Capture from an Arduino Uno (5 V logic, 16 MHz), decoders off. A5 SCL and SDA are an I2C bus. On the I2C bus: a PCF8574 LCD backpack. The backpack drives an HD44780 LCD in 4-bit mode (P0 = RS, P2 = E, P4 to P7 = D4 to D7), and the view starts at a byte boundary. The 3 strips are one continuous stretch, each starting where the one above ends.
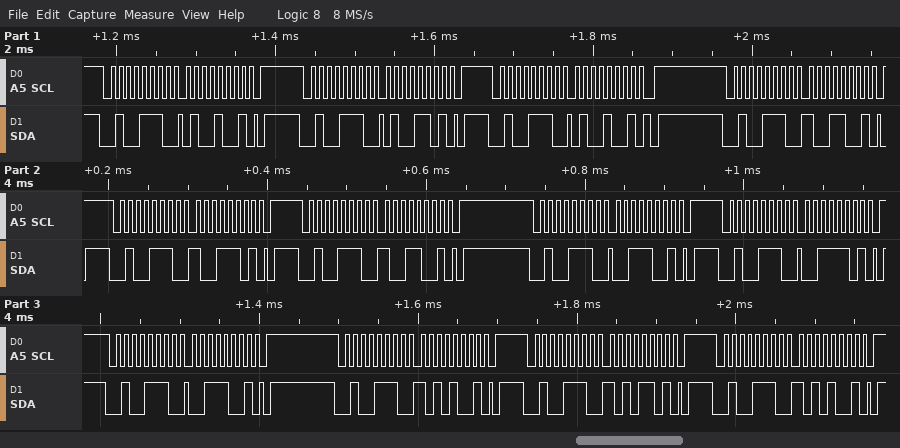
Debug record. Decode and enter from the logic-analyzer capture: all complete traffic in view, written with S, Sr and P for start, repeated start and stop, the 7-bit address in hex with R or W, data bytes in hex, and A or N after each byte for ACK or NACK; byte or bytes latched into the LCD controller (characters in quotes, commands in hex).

S 27W A 49 A P S 27W A 4D A P S 27W A 49 A P S 27W A 99 A P S 27W A 9D A P S 27W A 99 A P S 27W A 39 A P S 27W A 3D A P S 27W A 39 A P S 27W A A9 A P S 27W A AD A P S 27W A A9 A P
'I' ':'
